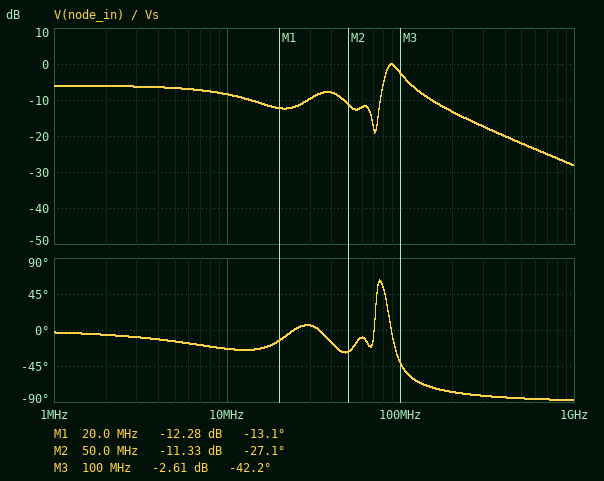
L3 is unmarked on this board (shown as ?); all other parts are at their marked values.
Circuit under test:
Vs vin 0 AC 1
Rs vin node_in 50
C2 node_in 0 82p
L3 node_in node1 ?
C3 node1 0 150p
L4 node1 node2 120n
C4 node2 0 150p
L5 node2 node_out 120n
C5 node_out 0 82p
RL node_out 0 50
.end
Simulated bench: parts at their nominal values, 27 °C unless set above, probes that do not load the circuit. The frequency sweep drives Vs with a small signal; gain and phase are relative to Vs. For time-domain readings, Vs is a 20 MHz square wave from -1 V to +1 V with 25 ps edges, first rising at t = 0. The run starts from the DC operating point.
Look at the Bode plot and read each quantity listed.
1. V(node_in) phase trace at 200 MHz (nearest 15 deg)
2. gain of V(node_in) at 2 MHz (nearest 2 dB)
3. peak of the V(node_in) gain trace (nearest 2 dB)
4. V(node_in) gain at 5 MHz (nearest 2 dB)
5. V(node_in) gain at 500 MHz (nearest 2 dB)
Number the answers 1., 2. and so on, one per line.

1. -75 deg
2. -6 dB
3. 0 dB
4. -6 dB
5. -22 dB
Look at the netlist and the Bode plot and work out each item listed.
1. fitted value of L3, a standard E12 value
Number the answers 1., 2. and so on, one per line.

1. 68 nH
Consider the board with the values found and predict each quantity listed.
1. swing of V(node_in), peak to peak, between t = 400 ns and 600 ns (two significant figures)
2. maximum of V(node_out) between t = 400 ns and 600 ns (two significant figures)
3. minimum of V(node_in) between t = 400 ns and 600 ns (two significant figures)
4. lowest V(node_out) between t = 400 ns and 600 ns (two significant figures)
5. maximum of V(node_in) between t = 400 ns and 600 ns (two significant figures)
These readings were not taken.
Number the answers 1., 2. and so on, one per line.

1. 870 mV
2. 570 mV
3. -430 mV
4. -570 mV
5. 430 mV
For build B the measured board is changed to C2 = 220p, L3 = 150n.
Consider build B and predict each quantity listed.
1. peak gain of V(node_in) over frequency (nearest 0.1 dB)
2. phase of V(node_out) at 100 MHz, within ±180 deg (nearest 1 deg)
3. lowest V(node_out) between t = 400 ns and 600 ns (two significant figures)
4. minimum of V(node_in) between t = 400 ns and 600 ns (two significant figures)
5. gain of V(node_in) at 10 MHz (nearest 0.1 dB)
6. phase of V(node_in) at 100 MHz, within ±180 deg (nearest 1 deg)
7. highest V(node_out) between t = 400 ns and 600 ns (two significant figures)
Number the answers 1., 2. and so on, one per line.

1. -6.0 dB
2. 128 deg
3. -590 mV
4. -400 mV
5. -9.4 dB
6. -81 deg
7. 590 mV
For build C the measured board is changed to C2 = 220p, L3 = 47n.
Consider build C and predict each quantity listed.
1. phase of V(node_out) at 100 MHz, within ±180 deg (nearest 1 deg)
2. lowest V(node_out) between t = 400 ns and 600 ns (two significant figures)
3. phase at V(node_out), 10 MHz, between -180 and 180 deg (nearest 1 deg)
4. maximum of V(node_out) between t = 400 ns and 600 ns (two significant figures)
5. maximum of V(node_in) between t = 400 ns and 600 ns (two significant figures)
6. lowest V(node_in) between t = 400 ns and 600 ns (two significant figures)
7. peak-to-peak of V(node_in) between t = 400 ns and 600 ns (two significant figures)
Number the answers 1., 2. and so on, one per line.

1. 134 deg
2. -460 mV
3. -56 deg
4. 460 mV
5. 340 mV
6. -340 mV
7. 680 mV
